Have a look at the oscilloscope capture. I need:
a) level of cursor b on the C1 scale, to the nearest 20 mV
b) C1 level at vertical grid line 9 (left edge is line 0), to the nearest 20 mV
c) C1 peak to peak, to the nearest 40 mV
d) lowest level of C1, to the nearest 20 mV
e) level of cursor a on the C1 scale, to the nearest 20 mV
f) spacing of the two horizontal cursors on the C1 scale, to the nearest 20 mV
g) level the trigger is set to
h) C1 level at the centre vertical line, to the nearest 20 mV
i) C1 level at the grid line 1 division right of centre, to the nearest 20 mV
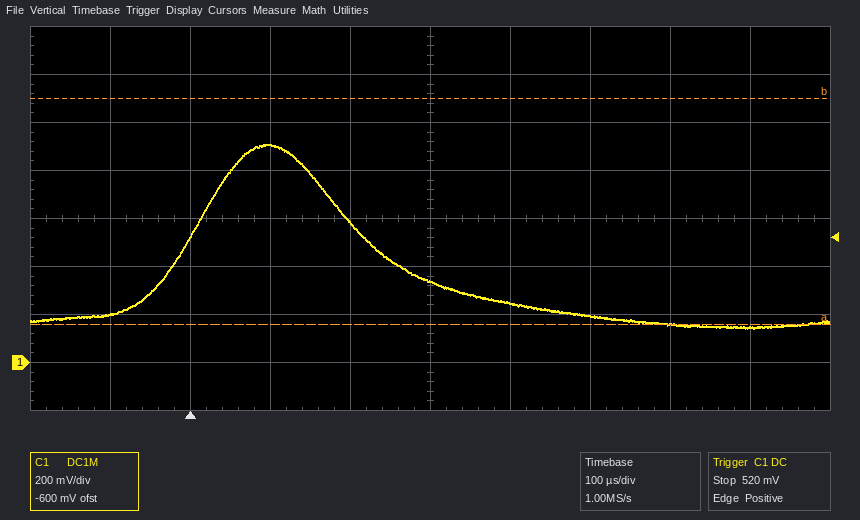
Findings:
1.10 V
140 mV
760 mV
140 mV
160 mV
940 mV
520 mV
340 mV
240 mV
